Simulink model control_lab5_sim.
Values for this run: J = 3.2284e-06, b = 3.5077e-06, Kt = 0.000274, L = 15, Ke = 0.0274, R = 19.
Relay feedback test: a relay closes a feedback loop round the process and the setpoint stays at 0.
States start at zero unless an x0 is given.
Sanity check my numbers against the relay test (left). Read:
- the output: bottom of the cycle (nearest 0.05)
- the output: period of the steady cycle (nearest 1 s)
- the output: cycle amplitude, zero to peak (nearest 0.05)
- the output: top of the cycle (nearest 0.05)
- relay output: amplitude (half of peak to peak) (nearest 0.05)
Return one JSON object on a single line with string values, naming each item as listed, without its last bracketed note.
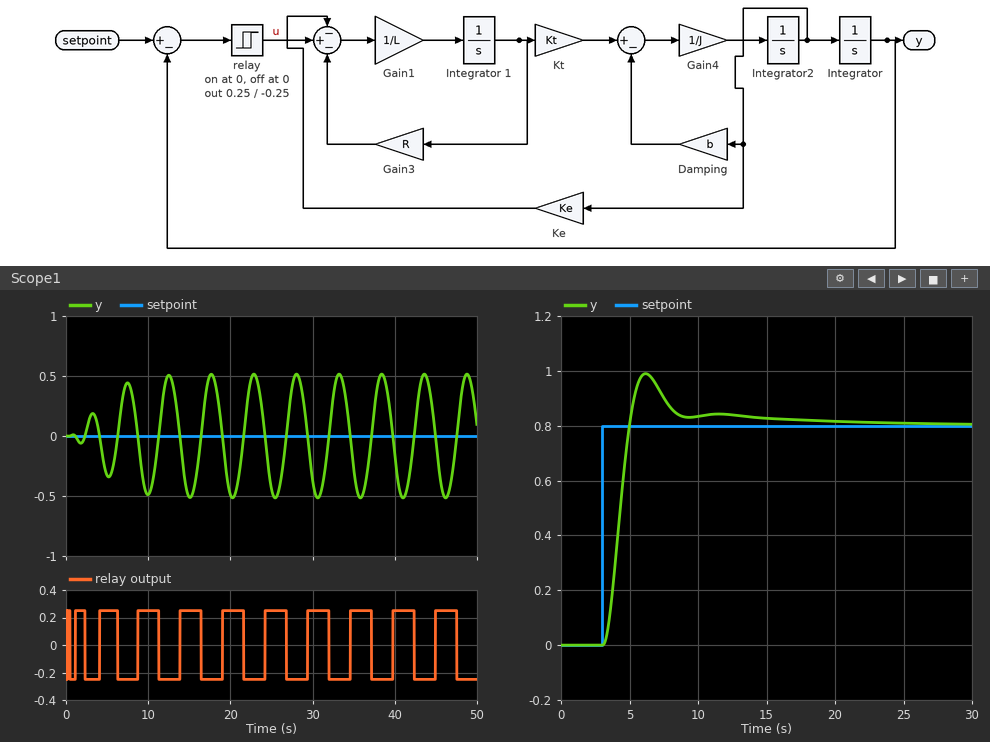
{"the output: bottom of the cycle": "-0.50", "the output: period of the steady cycle": "5 s", "the output: cycle amplitude, zero to peak": "0.50", "the output: top of the cycle": "0.50", "relay output: amplitude (half of peak to peak)": "0.25"}
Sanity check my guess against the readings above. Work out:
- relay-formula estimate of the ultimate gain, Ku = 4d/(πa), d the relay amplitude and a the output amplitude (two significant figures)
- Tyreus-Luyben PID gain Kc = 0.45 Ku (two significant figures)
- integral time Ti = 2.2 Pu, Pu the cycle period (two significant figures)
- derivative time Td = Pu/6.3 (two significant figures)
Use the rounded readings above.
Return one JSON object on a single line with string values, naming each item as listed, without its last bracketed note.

{"relay-formula estimate of the ultimate gain, Ku = 4d/(πa), d the relay amplitude and a the output amplitude": "0.64", "Tyreus-Luyben PID gain Kc = 0.45 Ku": "0.29", "integral time Ti = 2.2 Pu, Pu the cycle period": "11 s", "derivative time Td = Pu/6.3": "0.79 s"}
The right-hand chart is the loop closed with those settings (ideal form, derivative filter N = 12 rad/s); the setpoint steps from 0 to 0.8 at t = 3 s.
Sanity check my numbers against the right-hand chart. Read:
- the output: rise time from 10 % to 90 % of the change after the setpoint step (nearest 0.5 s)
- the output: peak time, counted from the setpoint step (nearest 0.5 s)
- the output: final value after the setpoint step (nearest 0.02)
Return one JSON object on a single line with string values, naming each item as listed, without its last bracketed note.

{"the output: rise time from 10 % to 90 % of the change after the setpoint step": "1.5 s", "the output: peak time, counted from the setpoint step": "3.0 s", "the output: final value after the setpoint step": "0.80"}
